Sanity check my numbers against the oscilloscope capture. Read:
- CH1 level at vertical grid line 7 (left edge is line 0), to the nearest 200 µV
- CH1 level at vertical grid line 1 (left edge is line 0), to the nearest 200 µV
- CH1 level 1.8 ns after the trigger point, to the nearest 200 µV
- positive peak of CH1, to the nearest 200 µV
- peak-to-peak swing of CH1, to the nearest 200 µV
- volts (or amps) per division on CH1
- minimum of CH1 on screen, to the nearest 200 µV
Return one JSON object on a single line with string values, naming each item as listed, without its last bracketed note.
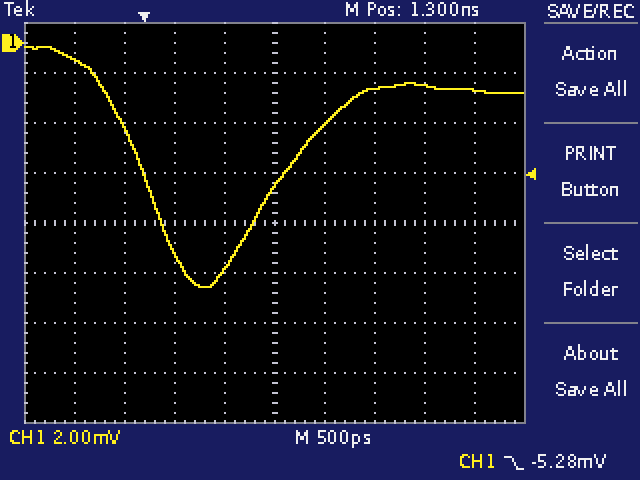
{"CH1 level at vertical grid line 7 (left edge is line 0), to the nearest 200 µV": "-1.8 mV", "CH1 level at vertical grid line 1 (left edge is line 0), to the nearest 200 µV": "-600 µV", "CH1 level 1.8 ns after the trigger point, to the nearest 200 µV": "-3.2 mV", "positive peak of CH1, to the nearest 200 µV": "-200 µV", "peak-to-peak swing of CH1, to the nearest 200 µV": "9.6 mV", "volts (or amps) per division on CH1": "2 mV", "minimum of CH1 on screen, to the nearest 200 µV": "-9.8 mV"}
